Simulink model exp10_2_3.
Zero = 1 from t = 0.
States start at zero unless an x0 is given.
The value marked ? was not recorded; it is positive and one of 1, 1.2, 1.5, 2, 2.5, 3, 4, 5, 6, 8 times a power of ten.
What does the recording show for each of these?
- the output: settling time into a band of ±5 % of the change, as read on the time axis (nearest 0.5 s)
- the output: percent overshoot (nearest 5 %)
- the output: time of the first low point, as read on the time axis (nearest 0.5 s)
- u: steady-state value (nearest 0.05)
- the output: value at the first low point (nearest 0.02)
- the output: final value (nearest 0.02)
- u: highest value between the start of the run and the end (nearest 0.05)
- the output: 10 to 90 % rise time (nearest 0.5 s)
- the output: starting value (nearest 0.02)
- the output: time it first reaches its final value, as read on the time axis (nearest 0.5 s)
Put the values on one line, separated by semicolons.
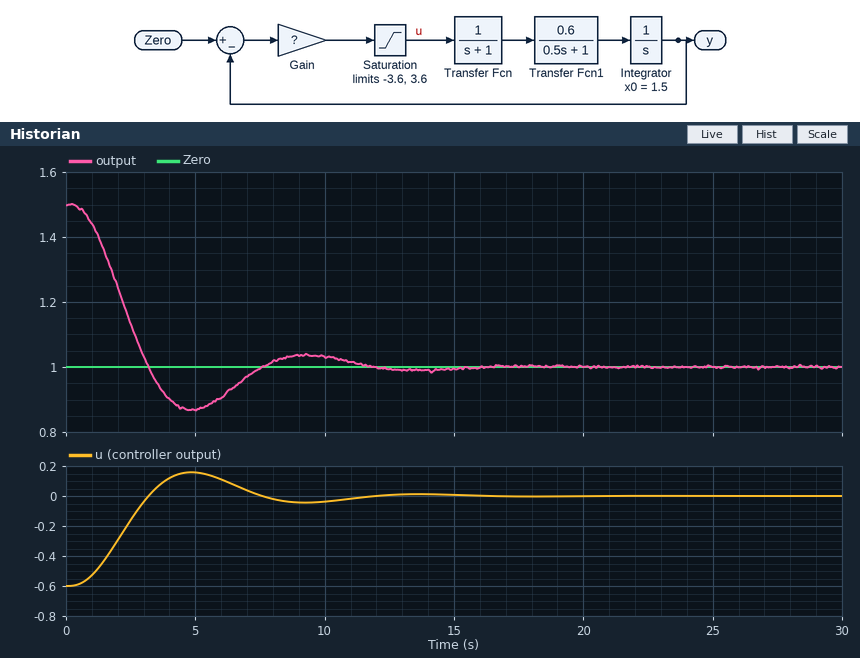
10.5 s; 25 %; 5.0 s; 0.00; 0.86; 1.00; 0.15; 2.0 s; 1.50; 3.0 s
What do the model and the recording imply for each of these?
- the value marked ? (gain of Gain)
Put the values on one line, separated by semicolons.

1.2
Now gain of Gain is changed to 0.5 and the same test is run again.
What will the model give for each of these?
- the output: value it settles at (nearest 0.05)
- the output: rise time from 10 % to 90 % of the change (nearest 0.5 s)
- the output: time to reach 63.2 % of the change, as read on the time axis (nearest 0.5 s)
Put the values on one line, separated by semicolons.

1.00; 4.5 s; 4.0 s
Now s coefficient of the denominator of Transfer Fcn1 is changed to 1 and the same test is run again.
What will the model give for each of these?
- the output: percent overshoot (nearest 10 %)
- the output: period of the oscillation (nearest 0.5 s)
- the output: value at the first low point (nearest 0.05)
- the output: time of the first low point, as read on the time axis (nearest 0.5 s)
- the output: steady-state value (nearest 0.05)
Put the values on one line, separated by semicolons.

40 %; 10.0 s; 0.80; 5.5 s; 1.00
